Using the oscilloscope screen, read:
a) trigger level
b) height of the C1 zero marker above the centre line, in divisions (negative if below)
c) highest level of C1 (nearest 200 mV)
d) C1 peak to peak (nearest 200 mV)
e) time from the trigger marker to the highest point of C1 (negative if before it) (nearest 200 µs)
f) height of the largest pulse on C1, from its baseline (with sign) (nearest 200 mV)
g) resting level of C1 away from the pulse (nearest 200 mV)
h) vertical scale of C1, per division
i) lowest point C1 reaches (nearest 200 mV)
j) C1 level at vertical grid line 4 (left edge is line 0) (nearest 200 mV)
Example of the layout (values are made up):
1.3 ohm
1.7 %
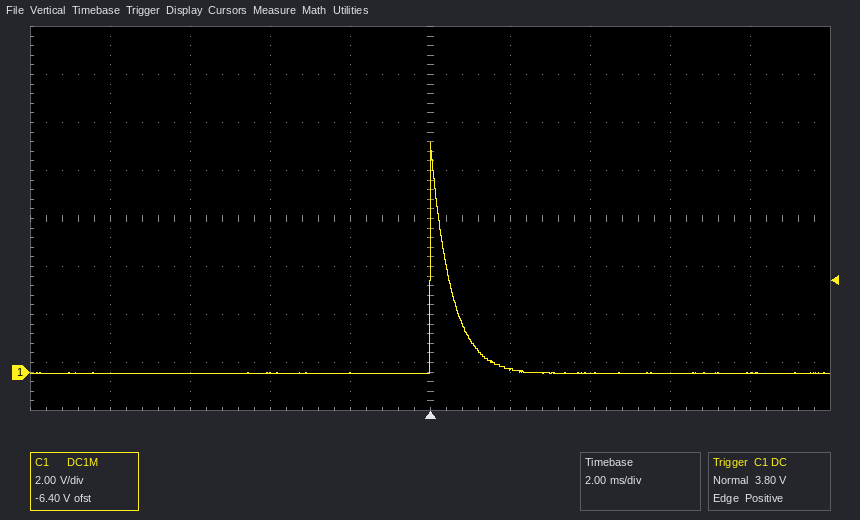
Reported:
3.80 V
-3.2 div
9.6 V
9.6 V
0.0 ms
+9.6 V
0.0 V
2 V
0.0 V
0.0 V
